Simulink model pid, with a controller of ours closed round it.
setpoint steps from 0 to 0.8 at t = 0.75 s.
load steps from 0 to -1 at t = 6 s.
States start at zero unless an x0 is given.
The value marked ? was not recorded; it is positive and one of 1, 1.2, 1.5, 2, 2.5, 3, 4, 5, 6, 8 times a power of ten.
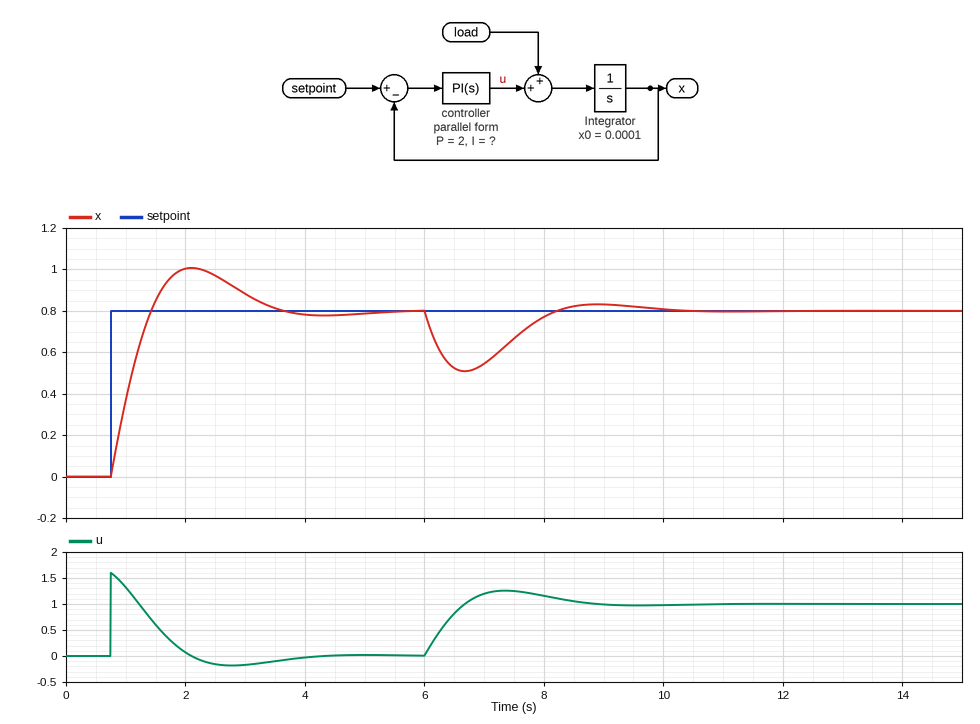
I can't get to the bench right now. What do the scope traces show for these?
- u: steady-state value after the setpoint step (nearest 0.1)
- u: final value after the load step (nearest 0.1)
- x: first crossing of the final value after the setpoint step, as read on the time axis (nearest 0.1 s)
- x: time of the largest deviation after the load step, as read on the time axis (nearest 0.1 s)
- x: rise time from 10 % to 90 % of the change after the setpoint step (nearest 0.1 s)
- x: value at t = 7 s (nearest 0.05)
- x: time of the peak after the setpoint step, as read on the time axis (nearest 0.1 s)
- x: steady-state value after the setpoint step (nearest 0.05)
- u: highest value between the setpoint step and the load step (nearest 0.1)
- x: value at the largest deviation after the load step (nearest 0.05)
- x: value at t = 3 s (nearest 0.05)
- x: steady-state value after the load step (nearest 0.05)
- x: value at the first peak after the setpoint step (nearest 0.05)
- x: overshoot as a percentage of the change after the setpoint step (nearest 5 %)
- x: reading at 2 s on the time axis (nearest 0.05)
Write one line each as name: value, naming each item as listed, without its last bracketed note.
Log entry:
u: steady-state value after the setpoint step: 0.0
u: final value after the load step: 1.0
x: first crossing of the final value after the setpoint step, as read on the time axis: 1.4 s
x: time of the largest deviation after the load step, as read on the time axis: 6.7 s
x: rise time from 10 % to 90 % of the change after the setpoint step: 0.5 s
x: value at t = 7 s: 0.55
x: time of the peak after the setpoint step, as read on the time axis: 2.1 s
x: steady-state value after the setpoint step: 0.80
u: highest value between the setpoint step and the load step: 1.6
x: value at the largest deviation after the load step: 0.50
x: value at t = 3 s: 0.90
x: steady-state value after the load step: 0.80
x: value at the first peak after the setpoint step: 1.00
x: overshoot as a percentage of the change after the setpoint step: 25 %
x: reading at 2 s on the time axis: 1.00
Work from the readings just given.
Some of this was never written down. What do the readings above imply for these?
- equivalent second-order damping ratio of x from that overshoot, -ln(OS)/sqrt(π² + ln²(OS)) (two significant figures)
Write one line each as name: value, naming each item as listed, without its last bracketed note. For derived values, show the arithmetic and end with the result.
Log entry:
equivalent second-order damping ratio of x from that overshoot, -ln(OS)/sqrt(π² + ln²(OS)): ln(0.25) = -1.386; 1.386 / sqrt(9.870 + 1.922) = 0.40
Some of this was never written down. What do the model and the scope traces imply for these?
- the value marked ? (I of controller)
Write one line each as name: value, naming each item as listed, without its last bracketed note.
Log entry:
the value marked ?: 3
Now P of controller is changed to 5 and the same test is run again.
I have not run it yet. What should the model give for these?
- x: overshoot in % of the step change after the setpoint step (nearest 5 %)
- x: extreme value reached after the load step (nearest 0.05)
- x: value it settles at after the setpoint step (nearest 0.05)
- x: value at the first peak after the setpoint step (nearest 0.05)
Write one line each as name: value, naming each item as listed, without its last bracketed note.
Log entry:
x: overshoot in % of the step change after the setpoint step: 10 %
x: extreme value reached after the load step: 0.65
x: value it settles at after the setpoint step: 0.80
x: value at the first peak after the setpoint step: 0.85
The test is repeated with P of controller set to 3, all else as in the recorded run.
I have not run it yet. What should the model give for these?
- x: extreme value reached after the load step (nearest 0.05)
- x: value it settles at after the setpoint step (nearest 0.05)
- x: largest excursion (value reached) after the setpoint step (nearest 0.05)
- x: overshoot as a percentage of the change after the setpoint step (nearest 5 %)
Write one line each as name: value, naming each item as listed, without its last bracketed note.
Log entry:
x: extreme value reached after the load step: 0.55
x: value it settles at after the setpoint step: 0.80
x: largest excursion (value reached) after the setpoint step: 0.95
x: overshoot as a percentage of the change after the setpoint step: 15 %
